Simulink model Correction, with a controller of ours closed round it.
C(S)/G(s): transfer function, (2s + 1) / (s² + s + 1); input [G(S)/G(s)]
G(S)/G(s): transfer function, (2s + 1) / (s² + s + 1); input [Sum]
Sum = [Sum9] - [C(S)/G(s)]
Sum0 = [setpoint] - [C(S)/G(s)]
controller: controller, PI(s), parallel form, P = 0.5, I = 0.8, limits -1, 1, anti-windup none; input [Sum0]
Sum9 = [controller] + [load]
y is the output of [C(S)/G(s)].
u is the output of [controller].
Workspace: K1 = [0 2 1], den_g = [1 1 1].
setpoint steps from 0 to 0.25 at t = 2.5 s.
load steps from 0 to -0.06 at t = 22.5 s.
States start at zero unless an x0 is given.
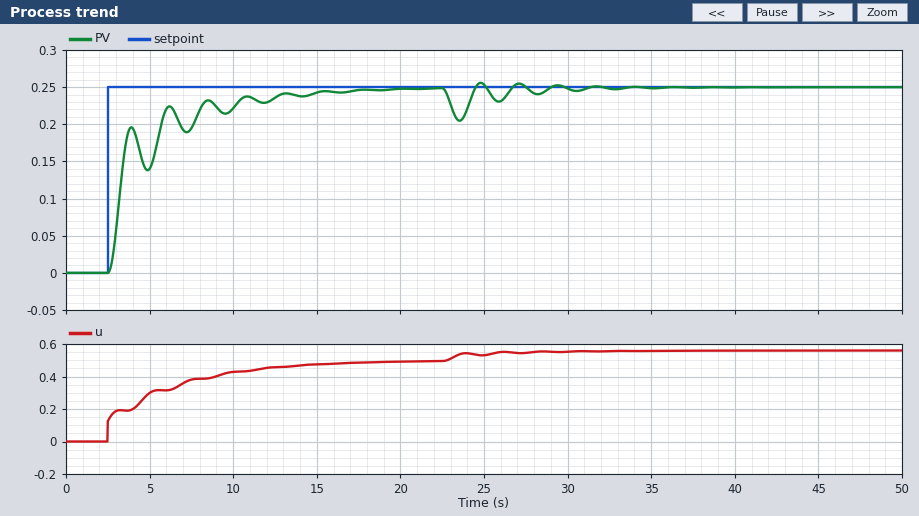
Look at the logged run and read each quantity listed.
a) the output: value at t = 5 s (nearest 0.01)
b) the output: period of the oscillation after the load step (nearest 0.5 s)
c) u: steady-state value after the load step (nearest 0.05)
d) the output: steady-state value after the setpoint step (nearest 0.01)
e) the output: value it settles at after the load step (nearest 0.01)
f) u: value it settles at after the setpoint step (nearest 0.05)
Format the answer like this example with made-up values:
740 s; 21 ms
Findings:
0.14; 2.5 s; 0.55; 0.25; 0.25; 0.50
